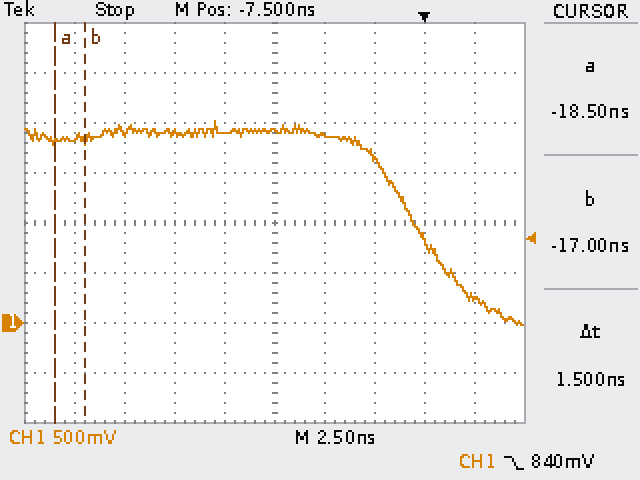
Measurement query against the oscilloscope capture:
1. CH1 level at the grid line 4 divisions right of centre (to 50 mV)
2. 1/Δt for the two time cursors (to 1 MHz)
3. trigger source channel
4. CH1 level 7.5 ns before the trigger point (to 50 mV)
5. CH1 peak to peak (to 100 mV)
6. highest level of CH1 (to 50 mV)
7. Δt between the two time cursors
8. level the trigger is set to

250 mV
667 MHz
CH1
1.90 V
2.00 V
2.00 V
1.5 ns
840 mV
